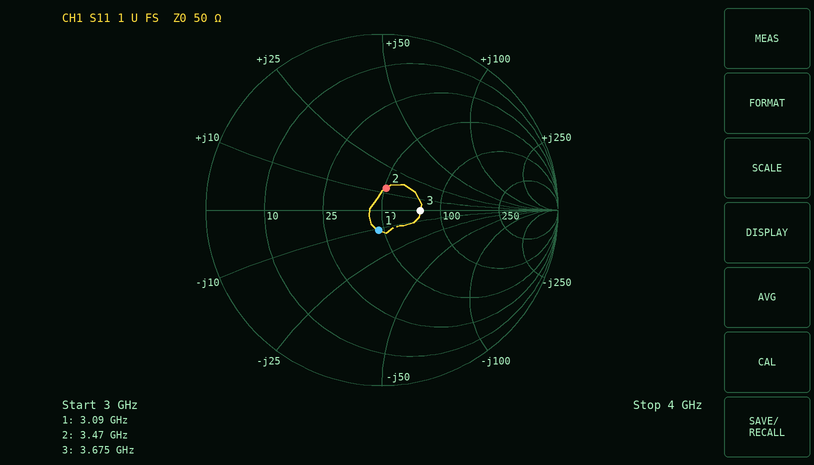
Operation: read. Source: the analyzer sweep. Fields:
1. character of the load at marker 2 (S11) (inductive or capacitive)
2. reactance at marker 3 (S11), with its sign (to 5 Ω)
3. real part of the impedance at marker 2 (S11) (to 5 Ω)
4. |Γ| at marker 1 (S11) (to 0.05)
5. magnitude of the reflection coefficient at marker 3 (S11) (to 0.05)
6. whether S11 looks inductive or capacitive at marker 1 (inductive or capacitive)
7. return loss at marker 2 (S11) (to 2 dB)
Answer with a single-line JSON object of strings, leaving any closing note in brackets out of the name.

{"character of the load at marker 2 (S11)": "inductive", "reactance at marker 3 (S11), with its sign": "0 Ω", "real part of the impedance at marker 2 (S11)": "50 Ω", "|Γ| at marker 1 (S11)": "0.10", "magnitude of the reflection coefficient at marker 3 (S11)": "0.20", "whether S11 looks inductive or capacitive at marker 1": "capacitive", "return loss at marker 2 (S11)": "18 dB"}
